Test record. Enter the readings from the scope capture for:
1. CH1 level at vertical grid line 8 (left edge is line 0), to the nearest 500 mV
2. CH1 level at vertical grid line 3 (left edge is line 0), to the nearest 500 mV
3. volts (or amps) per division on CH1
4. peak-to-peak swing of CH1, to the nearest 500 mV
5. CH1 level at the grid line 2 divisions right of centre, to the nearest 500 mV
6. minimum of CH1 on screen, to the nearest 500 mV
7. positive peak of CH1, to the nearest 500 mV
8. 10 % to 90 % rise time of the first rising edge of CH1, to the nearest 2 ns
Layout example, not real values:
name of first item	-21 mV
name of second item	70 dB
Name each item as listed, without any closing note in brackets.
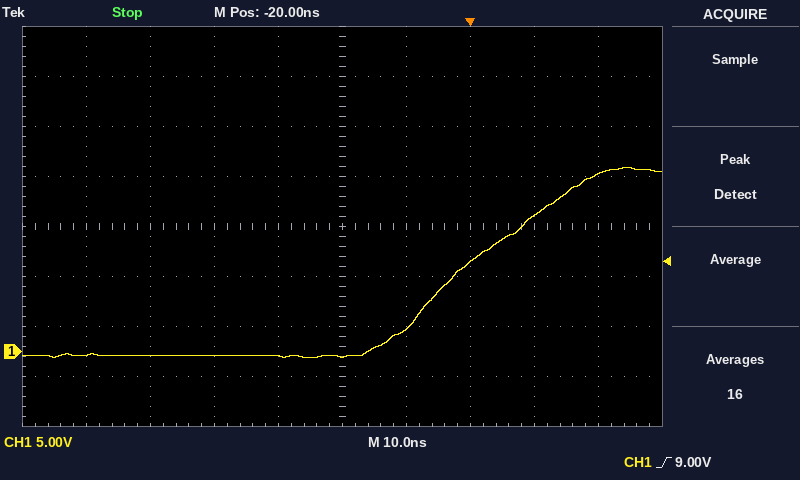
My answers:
CH1 level at vertical grid line 8 (left edge is line 0), to the nearest 500 mV	13.5 V
CH1 level at vertical grid line 3 (left edge is line 0), to the nearest 500 mV	-500 mV
volts (or amps) per division on CH1	5 V
peak-to-peak swing of CH1, to the nearest 500 mV	19.0 V
CH1 level at the grid line 2 divisions right of centre, to the nearest 500 mV	9.0 V
minimum of CH1 on screen, to the nearest 500 mV	-500 mV
positive peak of CH1, to the nearest 500 mV	18.5 V
10 % to 90 % rise time of the first rising edge of CH1, to the nearest 2 ns	28 ns
